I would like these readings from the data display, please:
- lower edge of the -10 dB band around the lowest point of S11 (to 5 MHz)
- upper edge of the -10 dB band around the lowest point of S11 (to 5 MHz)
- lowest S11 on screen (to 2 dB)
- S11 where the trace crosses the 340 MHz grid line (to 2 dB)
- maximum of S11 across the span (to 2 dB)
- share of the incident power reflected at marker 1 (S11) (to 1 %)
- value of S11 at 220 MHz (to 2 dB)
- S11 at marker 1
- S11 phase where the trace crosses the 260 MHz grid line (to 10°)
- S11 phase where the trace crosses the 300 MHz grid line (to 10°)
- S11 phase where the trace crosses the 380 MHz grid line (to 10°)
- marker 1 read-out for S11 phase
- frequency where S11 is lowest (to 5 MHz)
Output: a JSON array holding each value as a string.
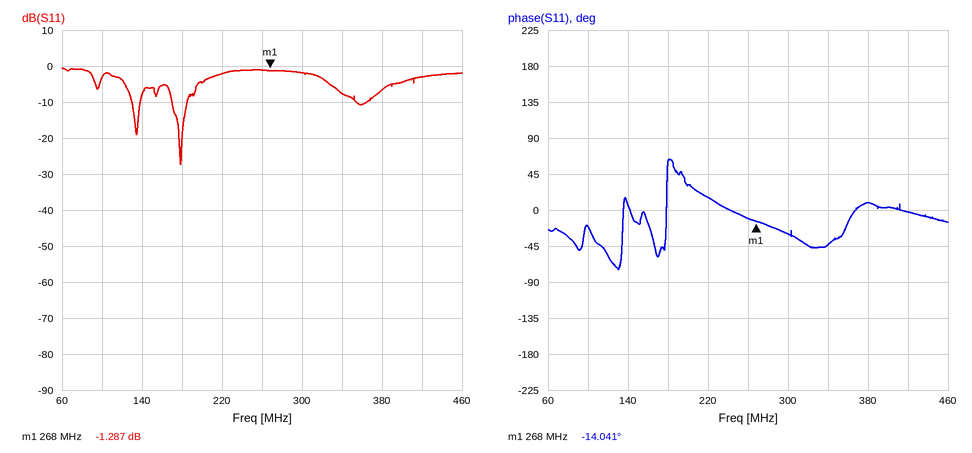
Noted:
["170 MHz", "185 MHz", "-28 dB", "-8 dB", "0 dB", "74 %", "-2 dB", "-1.287 dB", "-10°", "-30°", "10°", "-14.041°", "180 MHz"]
